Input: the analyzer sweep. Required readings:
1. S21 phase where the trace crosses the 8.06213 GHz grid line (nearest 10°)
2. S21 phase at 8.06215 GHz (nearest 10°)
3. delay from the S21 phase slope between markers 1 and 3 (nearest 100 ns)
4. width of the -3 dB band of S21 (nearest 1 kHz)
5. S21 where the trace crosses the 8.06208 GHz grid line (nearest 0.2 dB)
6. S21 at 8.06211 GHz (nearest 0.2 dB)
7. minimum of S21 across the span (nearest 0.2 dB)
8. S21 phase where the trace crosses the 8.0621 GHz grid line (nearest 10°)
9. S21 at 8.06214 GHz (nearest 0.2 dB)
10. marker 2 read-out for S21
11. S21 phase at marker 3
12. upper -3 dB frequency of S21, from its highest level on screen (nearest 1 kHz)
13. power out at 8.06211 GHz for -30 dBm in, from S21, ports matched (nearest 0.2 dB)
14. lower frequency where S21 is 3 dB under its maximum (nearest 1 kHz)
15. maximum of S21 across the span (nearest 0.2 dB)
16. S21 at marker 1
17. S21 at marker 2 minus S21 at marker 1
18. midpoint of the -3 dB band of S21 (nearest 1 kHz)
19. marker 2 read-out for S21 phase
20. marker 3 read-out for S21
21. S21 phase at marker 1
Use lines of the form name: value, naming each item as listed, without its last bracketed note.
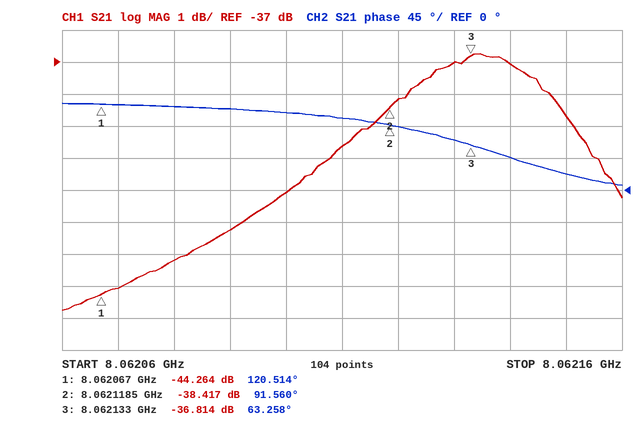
S21 phase where the trace crosses the 8.06213 GHz grid line: 70°
S21 phase at 8.06215 GHz: 20°
delay from the S21 phase slope between markers 1 and 3: 2.4 µs
width of the -3 dB band of S21: 45 kHz
S21 where the trace crosses the 8.06208 GHz grid line: -43.2 dB
S21 at 8.06211 GHz: -39.6 dB
minimum of S21 across the span: -44.8 dB
S21 phase where the trace crosses the 8.0621 GHz grid line: 110°
S21 at 8.06214 GHz: -37.0 dB
marker 2 read-out for S21: -38.417 dB
S21 phase at marker 3: 63.258°
upper -3 dB frequency of S21, from its highest level on screen: 8.062154 GHz
power out at 8.06211 GHz for -30 dBm in, from S21, ports matched: -69.6 dBm
lower frequency where S21 is 3 dB under its maximum: 8.062109 GHz
maximum of S21 across the span: -36.8 dB
S21 at marker 1: -44.264 dB
S21 at marker 2 minus S21 at marker 1: 5.847 dB
midpoint of the -3 dB band of S21: 8.062132 GHz
marker 2 read-out for S21 phase: 91.560°
marker 3 read-out for S21: -36.814 dB
S21 phase at marker 1: 120.514°
